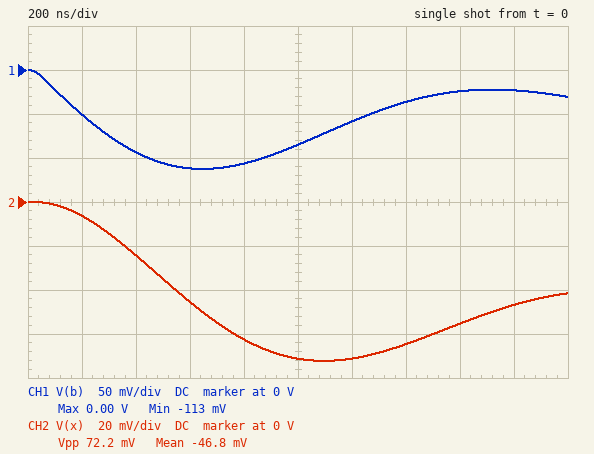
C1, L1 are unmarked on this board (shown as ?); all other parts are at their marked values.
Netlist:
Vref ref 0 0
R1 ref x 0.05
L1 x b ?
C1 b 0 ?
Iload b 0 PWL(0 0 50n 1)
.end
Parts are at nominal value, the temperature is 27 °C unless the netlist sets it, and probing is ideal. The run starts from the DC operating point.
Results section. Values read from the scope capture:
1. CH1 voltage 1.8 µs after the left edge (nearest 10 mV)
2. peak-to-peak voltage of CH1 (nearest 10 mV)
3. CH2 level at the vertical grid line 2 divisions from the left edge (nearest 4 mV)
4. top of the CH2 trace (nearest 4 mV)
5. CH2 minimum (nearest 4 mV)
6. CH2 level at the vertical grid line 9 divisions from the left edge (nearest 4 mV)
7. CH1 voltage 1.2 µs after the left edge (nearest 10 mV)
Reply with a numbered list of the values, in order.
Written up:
1. -20 mV
2. 110 mV
3. -24 mV
4. 0 V
5. -72 mV
6. -48 mV
7. -60 mV
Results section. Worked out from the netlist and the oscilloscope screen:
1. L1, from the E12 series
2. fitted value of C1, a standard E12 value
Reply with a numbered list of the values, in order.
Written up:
1. 33 nH
2. 3.3 µF
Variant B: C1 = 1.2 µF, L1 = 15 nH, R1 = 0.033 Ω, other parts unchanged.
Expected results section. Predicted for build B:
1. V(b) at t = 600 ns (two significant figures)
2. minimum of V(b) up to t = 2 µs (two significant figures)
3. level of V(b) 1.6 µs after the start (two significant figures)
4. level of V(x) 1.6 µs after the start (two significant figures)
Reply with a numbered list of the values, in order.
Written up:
1. 9.8 mV
2. -120 mV
3. -14 mV
4. -30 mV
